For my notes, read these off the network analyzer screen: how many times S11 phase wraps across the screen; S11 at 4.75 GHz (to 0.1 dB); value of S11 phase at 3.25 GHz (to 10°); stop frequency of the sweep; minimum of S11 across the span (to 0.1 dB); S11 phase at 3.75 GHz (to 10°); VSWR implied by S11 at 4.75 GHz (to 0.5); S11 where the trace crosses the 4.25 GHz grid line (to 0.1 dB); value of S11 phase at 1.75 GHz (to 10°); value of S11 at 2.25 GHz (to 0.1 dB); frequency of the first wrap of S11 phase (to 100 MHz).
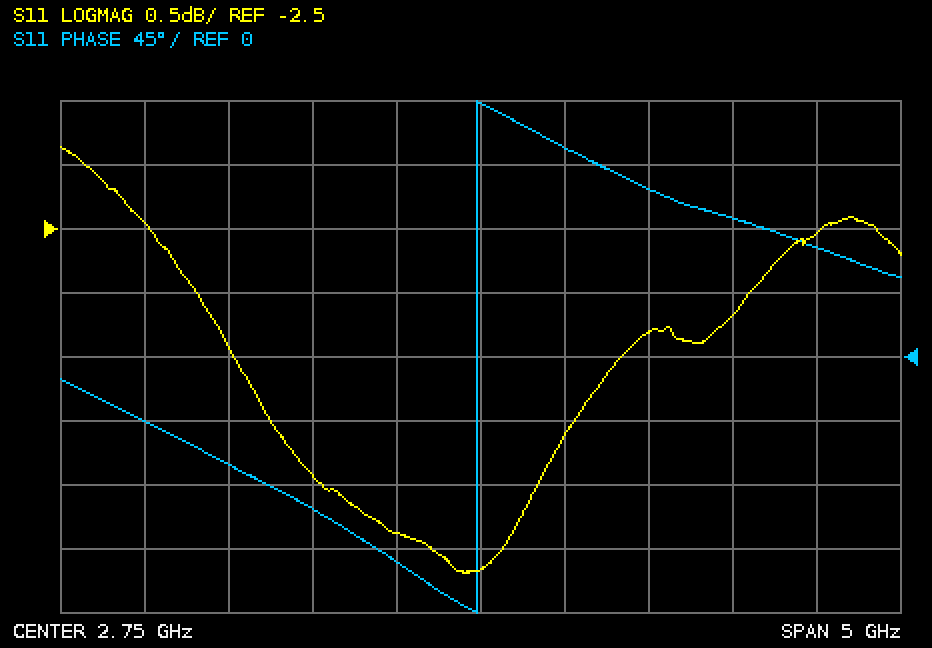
1
-2.5 dB
150°
5.25 GHz
-5.2 dB
120°
7.0
-3.2 dB
-110°
-4.9 dB
2.7 GHz
